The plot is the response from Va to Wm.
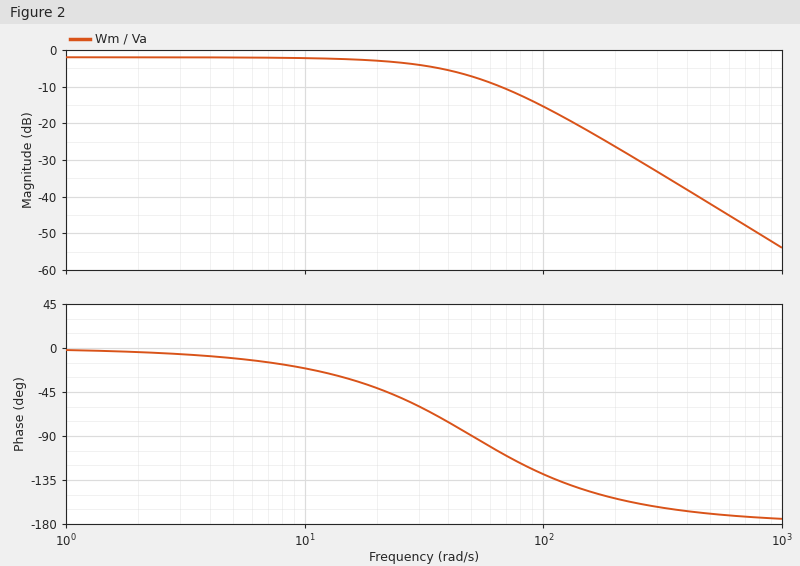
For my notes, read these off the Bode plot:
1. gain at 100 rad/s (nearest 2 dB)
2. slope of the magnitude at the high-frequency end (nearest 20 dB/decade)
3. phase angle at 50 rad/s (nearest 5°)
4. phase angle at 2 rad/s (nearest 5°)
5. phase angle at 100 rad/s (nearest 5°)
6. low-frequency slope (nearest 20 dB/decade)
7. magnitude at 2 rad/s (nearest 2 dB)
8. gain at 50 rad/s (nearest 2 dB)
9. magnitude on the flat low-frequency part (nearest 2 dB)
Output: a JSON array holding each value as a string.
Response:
["-16 dB", "-40 dB/decade", "-90°", "-5°", "-130°", "0 dB/decade", "-2 dB", "-8 dB", "-2 dB"]
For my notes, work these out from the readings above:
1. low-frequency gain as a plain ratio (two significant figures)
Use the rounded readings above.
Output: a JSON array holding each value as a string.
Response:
["0.79"]
